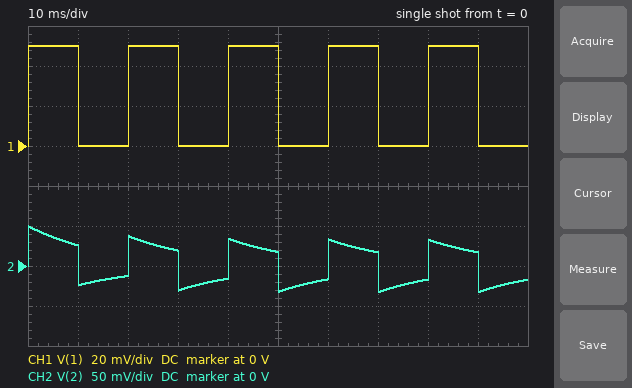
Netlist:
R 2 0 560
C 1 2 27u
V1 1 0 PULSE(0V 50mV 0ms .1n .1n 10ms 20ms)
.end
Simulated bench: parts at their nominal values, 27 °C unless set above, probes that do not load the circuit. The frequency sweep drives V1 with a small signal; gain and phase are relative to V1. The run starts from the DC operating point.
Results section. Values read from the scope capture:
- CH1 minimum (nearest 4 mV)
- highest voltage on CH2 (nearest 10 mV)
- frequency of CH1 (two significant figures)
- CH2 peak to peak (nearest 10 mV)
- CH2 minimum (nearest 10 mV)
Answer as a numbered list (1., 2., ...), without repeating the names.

1. 0 V
2. 50 mV
3. 50 Hz
4. 80 mV
5. -30 mV
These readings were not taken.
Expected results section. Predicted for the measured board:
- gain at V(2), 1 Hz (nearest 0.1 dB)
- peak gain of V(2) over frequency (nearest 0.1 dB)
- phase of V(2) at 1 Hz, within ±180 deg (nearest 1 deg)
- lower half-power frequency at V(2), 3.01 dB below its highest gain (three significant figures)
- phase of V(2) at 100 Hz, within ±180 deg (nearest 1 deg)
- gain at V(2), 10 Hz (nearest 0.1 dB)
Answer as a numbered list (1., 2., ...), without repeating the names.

1. -20.5 dB
2. 0 dB
3. 85 deg
4. 10.5 Hz
5. 6 deg
6. -3.2 dB
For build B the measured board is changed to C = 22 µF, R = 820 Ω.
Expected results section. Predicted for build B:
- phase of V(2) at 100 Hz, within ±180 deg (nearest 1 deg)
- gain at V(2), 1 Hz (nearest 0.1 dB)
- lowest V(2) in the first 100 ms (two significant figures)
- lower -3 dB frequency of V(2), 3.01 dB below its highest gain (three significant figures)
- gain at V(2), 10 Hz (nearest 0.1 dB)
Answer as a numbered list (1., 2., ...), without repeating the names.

1. 5 deg
2. -19.0 dB
3. -32 mV
4. 8.82 Hz
5. -2.5 dB
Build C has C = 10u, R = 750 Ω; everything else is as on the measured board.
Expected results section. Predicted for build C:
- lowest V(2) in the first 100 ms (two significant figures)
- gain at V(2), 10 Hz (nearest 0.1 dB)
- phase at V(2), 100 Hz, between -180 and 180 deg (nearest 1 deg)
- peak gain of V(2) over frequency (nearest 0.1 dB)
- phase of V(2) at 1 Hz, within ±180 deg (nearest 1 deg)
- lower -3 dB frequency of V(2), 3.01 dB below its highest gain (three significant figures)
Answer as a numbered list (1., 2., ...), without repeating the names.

1. -40 mV
2. -7.4 dB
3. 12 deg
4. 0 dB
5. 87 deg
6. 21.2 Hz
